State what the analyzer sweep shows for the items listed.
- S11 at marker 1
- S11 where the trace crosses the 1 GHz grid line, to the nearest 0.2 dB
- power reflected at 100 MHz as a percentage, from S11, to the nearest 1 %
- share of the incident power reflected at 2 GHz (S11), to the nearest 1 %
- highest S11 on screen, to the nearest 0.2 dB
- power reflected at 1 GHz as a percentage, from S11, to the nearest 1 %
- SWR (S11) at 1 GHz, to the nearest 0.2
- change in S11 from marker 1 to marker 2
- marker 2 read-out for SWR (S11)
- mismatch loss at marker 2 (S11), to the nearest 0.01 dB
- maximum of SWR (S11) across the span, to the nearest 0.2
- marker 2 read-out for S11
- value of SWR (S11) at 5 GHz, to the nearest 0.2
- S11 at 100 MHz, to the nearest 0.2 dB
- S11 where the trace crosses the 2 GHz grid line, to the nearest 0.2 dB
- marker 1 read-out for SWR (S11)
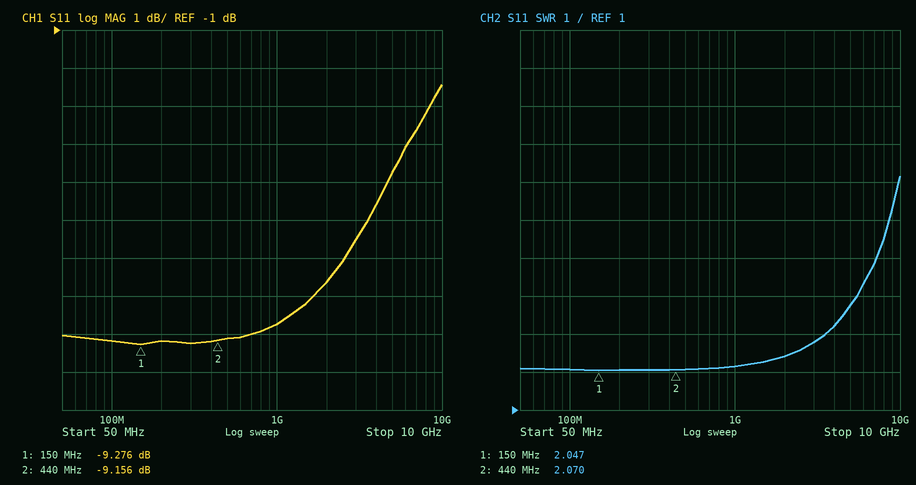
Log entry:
-9.276 dB
-8.8 dB
12 %
17 %
-2.4 dB
13 %
2.2
0.120 dB
2.070
0.56 dB
7.2
-9.156 dB
3.8
-9.2 dB
-7.6 dB
2.047
